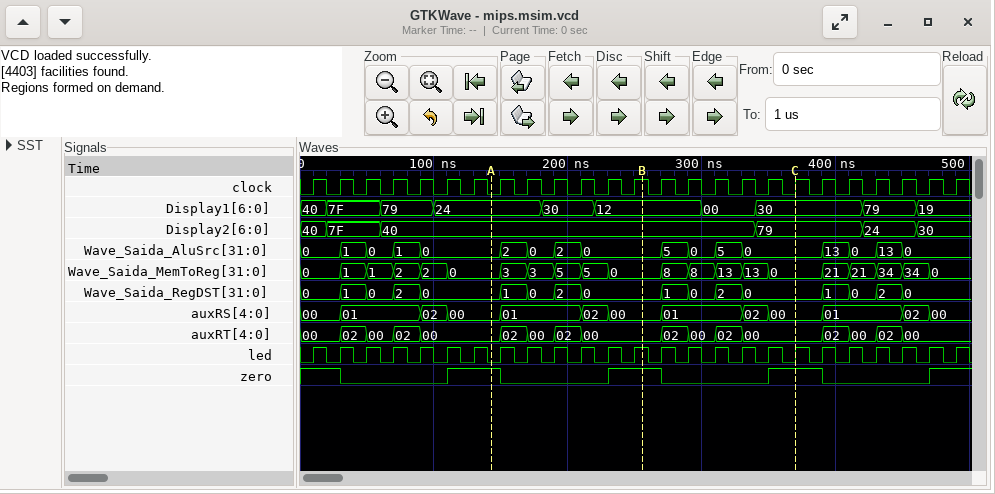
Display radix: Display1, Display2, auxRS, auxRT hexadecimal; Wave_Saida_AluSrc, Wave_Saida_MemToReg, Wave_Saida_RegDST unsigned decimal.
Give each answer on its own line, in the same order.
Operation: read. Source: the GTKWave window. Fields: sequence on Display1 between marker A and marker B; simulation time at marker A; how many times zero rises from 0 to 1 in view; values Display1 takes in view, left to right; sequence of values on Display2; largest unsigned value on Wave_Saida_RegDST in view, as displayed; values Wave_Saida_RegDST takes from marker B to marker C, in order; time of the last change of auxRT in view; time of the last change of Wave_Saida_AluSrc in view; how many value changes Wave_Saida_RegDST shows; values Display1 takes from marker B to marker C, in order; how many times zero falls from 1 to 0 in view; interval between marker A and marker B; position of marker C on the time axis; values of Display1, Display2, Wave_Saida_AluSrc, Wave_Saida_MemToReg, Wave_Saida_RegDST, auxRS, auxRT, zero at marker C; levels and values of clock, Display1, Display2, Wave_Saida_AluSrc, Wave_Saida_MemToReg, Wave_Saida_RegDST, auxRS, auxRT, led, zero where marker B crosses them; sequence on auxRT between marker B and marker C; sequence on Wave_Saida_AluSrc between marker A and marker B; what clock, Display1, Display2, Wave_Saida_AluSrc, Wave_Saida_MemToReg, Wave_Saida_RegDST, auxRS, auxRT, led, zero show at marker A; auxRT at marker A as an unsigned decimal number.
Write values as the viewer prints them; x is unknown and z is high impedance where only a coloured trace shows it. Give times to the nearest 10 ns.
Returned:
24, 30, 12
140 ns
4
40, 7F, 79, 24, 30, 12, 00, 30, 79, 19
40, 7F, 40, 79, 24, 30
2
0, 1, 0, 2, 0
450 ns
450 ns
16
12, 00, 30
4
110 ns
370 ns
Display1=30, Display2=79, Wave_Saida_AluSrc=0, Wave_Saida_MemToReg=0, Wave_Saida_RegDST=0, auxRS=00, auxRT=00, zero=1
clock=1, Display1=12, Display2=40, Wave_Saida_AluSrc=0, Wave_Saida_MemToReg=0, Wave_Saida_RegDST=0, auxRS=00, auxRT=00, led=1, zero=1
00, 02, 00, 02, 00
0, 2, 0, 2, 0
clock=0, Display1=24, Display2=40, Wave_Saida_AluSrc=0, Wave_Saida_MemToReg=0, Wave_Saida_RegDST=0, auxRS=00, auxRT=00, led=0, zero=1
0
